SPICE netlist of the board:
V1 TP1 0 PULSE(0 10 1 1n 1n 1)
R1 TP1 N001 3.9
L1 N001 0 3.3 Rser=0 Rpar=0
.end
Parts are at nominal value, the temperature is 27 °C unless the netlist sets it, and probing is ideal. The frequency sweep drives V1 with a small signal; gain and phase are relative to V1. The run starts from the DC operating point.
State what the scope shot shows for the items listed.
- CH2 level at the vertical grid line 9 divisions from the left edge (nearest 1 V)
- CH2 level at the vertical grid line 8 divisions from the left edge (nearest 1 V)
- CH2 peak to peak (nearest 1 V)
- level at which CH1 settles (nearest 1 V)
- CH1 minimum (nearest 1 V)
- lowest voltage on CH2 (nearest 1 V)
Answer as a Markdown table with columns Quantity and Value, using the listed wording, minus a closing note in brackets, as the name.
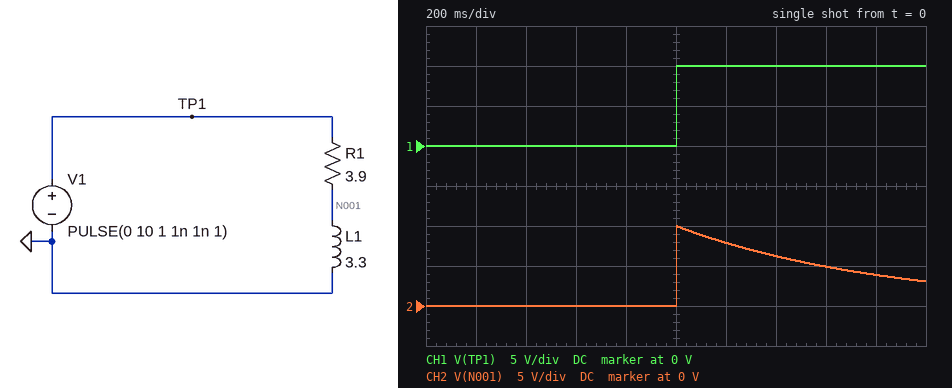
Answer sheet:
| Quantity | Value |
|---|---|
| CH2 level at the vertical grid line 9 divisions from the left edge | 4 V |
| CH2 level at the vertical grid line 8 divisions from the left edge | 5 V |
| CH2 peak to peak | 10 V |
| level at which CH1 settles | 10 V |
| CH1 minimum | 0 V |
| lowest voltage on CH2 | 0 V |
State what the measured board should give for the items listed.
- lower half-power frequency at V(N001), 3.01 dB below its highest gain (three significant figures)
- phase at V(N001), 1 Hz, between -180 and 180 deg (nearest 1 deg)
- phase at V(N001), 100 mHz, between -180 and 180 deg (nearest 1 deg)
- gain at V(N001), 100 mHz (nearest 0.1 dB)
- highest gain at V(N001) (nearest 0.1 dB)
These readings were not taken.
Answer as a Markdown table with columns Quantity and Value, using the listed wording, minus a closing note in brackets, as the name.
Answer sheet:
| Quantity | Value |
|---|---|
| lower half-power frequency at V(N001), 3.01 dB below its highest gain | 188 mHz |
| phase at V(N001), 1 Hz, between -180 and 180 deg | 11 deg |
| phase at V(N001), 100 mHz, between -180 and 180 deg | 62 deg |
| gain at V(N001), 100 mHz | -6.6 dB |
| highest gain at V(N001) | 0 dB |
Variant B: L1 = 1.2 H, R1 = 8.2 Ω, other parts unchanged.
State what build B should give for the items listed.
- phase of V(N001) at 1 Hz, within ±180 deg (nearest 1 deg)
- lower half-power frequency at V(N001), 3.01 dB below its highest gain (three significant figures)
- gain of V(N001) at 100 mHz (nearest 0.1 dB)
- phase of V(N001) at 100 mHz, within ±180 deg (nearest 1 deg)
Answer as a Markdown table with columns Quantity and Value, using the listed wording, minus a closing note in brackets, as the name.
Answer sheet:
| Quantity | Value |
|---|---|
| phase of V(N001) at 1 Hz, within ±180 deg | 47 deg |
| lower half-power frequency at V(N001), 3.01 dB below its highest gain | 1.09 Hz |
| gain of V(N001) at 100 mHz | -20.8 dB |
| phase of V(N001) at 100 mHz, within ±180 deg | 85 deg |
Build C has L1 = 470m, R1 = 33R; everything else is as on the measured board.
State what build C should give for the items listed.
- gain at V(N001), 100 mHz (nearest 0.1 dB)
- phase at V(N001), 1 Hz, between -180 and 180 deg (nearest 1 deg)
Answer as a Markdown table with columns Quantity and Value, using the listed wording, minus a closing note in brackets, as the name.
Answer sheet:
| Quantity | Value |
|---|---|
| gain at V(N001), 100 mHz | -41.0 dB |
| phase at V(N001), 1 Hz, between -180 and 180 deg | 85 deg |
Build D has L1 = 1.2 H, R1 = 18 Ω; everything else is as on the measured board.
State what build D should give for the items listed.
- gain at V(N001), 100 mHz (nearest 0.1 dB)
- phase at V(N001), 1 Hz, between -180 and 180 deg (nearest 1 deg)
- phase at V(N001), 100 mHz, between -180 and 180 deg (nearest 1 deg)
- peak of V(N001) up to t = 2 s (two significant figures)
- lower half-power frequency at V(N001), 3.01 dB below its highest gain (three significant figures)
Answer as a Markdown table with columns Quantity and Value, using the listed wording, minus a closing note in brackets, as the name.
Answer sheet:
| Quantity | Value |
|---|---|
| gain at V(N001), 100 mHz | -27.6 dB |
| phase at V(N001), 1 Hz, between -180 and 180 deg | 67 deg |
| phase at V(N001), 100 mHz, between -180 and 180 deg | 88 deg |
| peak of V(N001) up to t = 2 s | 10 V |
| lower half-power frequency at V(N001), 3.01 dB below its highest gain | 2.39 Hz |
